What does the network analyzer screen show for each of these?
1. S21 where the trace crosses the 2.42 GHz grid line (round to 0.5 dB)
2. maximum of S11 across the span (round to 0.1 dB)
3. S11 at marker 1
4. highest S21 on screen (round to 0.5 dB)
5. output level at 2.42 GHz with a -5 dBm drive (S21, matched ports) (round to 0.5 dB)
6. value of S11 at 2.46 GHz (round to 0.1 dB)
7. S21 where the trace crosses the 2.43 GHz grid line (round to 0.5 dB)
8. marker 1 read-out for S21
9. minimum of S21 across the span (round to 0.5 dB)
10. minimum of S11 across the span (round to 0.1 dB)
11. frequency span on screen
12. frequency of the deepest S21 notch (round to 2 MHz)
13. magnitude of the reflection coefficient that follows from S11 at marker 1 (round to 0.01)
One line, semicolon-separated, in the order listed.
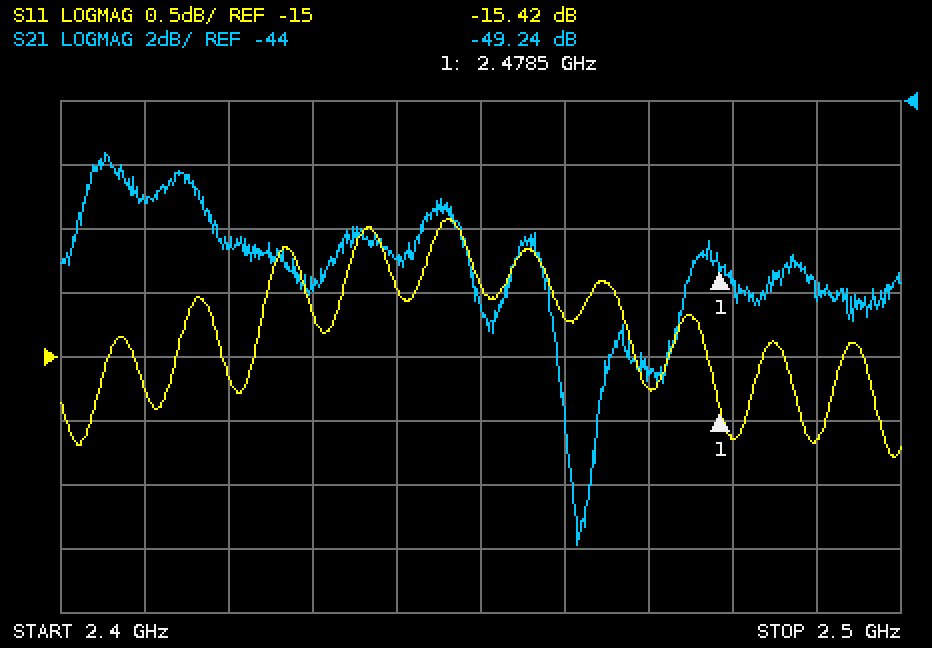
-48.5 dB; -13.9 dB; -15.42 dB; -45.5 dB; -53.5 dBm; -14.7 dB; -50.0 dB; -49.24 dB; -58.0 dB; -15.8 dB; 100 MHz; 2.462 GHz; 0.17
